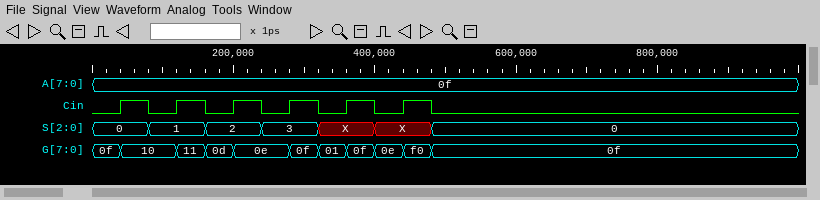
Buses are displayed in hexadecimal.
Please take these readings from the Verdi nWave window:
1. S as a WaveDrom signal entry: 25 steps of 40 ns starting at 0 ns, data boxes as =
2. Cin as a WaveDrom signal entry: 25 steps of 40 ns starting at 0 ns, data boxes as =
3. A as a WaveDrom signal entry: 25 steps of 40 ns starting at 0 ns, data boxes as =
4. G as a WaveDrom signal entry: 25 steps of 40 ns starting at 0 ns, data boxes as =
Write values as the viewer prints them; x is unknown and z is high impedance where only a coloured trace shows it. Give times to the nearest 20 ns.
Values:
{name: 'S', wave: '=.=.=.=.=.=.=............', data: '0 1 2 3 X X 0'}
{name: 'Cin', wave: '0101010101010............'}
{name: 'A', wave: '=........................', data: '0f'}
{name: 'G', wave: '==.===.======............', data: '0f 10 11 0d 0e 0f 01 0f 0e f0 0f'}
